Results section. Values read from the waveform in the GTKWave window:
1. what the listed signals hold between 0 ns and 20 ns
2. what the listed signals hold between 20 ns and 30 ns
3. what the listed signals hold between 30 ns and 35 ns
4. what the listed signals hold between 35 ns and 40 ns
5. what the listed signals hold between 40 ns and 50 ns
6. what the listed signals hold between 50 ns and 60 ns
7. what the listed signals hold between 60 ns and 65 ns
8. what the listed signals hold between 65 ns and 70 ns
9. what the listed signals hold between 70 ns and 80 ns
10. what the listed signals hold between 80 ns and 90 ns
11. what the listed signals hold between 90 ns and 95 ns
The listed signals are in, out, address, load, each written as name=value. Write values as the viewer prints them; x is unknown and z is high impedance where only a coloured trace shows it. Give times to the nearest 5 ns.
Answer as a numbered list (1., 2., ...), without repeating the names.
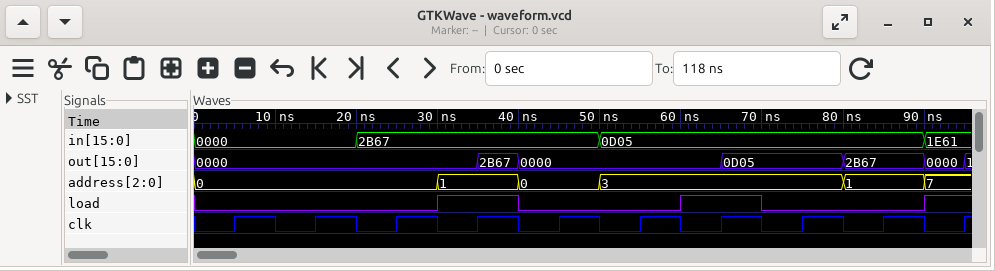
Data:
1. in=0000, out=0000, address=0, load=0
2. in=2B67, out=0000, address=0, load=0
3. in=2B67, out=0000, address=1, load=1
4. in=2B67, out=2B67, address=1, load=1
5. in=2B67, out=0000, address=0, load=0
6. in=0D05, out=0000, address=3, load=0
7. in=0D05, out=0000, address=3, load=1
8. in=0D05, out=0D05, address=3, load=1
9. in=0D05, out=0D05, address=3, load=0
10. in=0D05, out=2B67, address=1, load=0
11. in=1E61, out=0000, address=7, load=1
